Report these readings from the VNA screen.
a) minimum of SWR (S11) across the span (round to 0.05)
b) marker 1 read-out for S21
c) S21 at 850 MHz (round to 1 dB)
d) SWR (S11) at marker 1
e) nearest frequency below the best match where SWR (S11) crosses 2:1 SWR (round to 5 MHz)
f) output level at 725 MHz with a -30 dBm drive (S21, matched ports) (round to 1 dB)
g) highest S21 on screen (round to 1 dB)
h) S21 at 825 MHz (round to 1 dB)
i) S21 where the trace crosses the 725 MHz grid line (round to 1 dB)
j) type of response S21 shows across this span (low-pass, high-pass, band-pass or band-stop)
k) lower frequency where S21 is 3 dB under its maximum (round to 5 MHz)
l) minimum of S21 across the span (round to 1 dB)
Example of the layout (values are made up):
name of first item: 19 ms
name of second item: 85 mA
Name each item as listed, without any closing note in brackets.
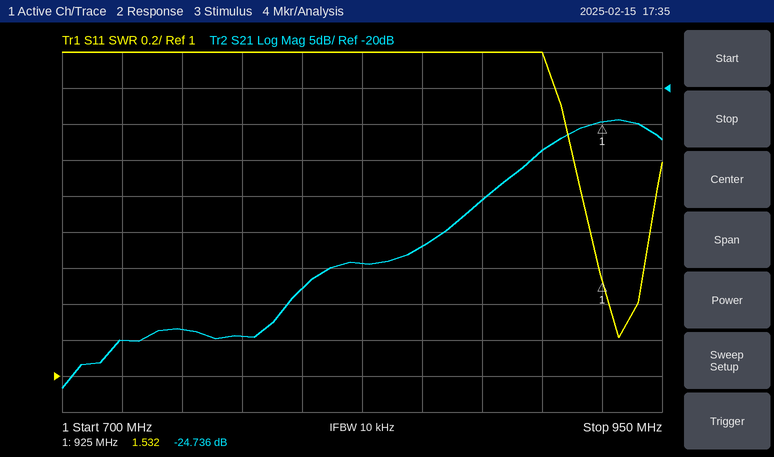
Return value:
minimum of SWR (S11) across the span: 1.20
marker 1 read-out for S21: -24.736 dB
S21 at 850 MHz: -42 dB
SWR (S11) at marker 1: 1.532
nearest frequency below the best match where SWR (S11) crosses 2:1 SWR: 915 MHz
output level at 725 MHz with a -30 dBm drive (S21, matched ports): -85 dBm
highest S21 on screen: -24 dB
S21 at 825 MHz: -44 dB
S21 where the trace crosses the 725 MHz grid line: -55 dB
type of response S21 shows across this span: high-pass
lower frequency where S21 is 3 dB under its maximum: 905 MHz
minimum of S21 across the span: -62 dB
